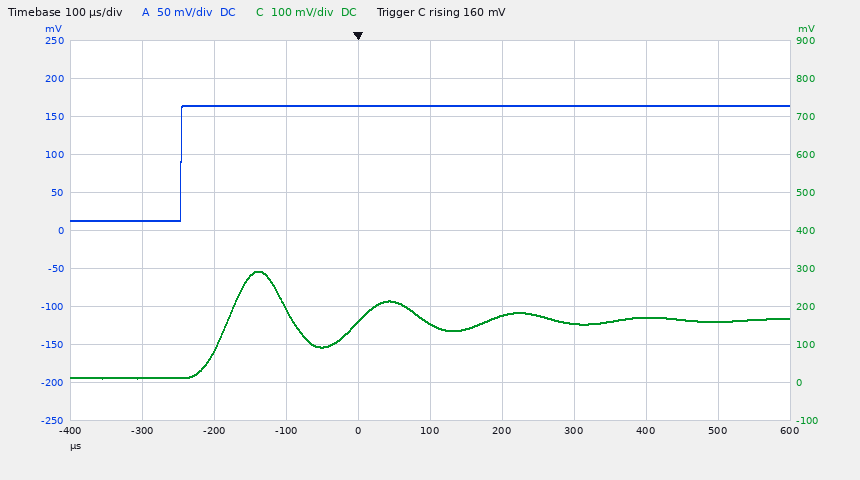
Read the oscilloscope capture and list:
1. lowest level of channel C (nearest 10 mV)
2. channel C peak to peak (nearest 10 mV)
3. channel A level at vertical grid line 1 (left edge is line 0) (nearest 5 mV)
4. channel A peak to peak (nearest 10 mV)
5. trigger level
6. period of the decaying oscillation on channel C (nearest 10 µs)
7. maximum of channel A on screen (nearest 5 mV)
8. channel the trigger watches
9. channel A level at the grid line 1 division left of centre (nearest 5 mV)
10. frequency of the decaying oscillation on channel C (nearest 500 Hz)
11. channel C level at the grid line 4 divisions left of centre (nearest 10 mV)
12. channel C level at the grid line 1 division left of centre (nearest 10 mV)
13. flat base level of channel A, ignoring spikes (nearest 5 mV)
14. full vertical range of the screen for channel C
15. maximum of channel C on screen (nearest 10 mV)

10 mV
280 mV
15 mV
150 mV
160 mV
180 µs
165 mV
channel C
165 mV
5.5 kHz
10 mV
160 mV
15 mV
1 V
290 mV
